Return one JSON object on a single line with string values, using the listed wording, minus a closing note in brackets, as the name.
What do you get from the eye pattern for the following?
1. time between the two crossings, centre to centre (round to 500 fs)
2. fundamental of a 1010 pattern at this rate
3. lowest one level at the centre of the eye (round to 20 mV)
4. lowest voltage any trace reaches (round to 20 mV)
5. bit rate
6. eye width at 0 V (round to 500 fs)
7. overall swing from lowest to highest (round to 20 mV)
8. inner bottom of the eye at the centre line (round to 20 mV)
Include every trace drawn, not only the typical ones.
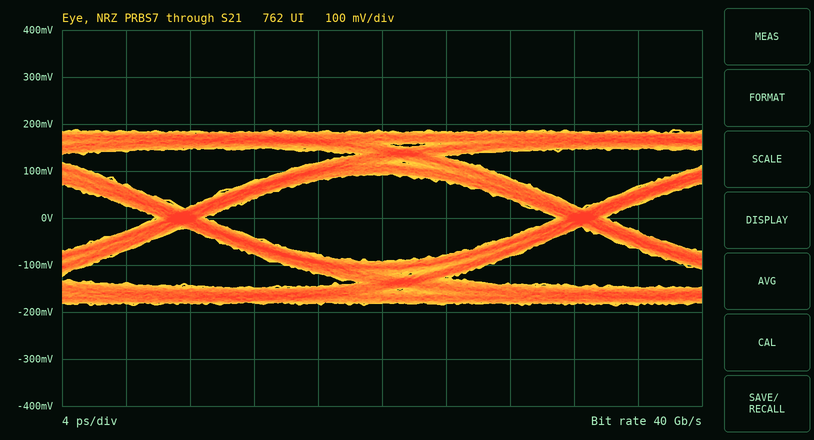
{"time between the two crossings, centre to centre": "25.0 ps", "fundamental of a 1010 pattern at this rate": "20 GHz", "lowest one level at the centre of the eye": "100 mV", "lowest voltage any trace reaches": "-180 mV", "bit rate": "40 Gb/s", "eye width at 0 V": "22.0 ps", "overall swing from lowest to highest": "380 mV", "inner bottom of the eye at the centre line": "-100 mV"}
